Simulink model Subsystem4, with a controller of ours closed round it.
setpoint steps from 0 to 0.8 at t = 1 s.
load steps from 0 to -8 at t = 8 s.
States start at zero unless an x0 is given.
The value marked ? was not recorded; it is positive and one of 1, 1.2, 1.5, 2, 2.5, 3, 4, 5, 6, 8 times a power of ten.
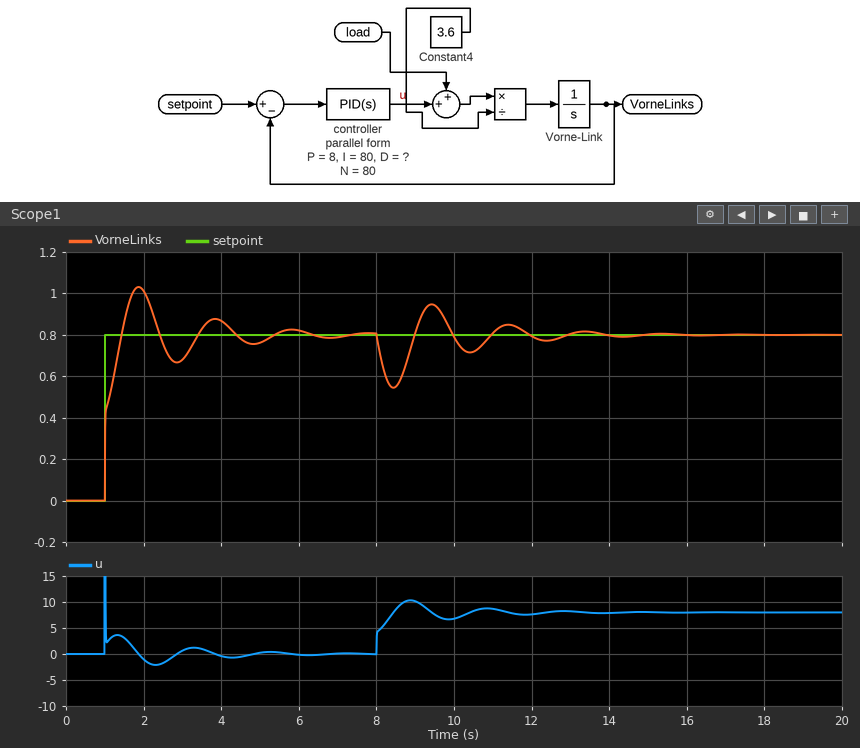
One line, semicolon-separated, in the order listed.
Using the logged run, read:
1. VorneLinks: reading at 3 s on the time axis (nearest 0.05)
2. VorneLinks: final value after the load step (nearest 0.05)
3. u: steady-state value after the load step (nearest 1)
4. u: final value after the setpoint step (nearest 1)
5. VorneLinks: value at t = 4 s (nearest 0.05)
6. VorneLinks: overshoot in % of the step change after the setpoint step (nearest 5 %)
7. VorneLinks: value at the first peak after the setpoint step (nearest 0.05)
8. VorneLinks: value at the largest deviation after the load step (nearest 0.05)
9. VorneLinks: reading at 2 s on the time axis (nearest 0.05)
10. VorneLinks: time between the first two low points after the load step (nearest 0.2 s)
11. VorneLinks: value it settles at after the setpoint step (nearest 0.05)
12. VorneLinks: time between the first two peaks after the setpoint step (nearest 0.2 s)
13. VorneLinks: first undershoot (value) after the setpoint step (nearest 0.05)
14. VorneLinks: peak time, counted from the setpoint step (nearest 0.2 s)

0.70; 0.80; 8; 0; 0.85; 30 %; 1.05; 0.55; 1.00; 2.0 s; 0.80; 2.0 s; 0.65; 0.8 s
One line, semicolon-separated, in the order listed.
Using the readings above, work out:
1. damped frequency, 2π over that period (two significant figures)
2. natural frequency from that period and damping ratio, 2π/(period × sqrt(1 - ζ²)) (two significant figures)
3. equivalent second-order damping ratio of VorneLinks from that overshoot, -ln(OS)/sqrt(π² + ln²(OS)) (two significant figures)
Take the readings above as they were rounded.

3.1 rad/s; 3.4 rad/s; 0.36
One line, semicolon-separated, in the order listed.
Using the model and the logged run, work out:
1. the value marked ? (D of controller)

4
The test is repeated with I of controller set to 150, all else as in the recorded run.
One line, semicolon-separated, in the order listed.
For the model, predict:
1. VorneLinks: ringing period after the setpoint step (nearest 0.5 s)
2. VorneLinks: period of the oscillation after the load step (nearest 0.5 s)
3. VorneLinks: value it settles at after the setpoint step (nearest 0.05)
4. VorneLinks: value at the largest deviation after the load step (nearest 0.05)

1.5 s; 1.5 s; 0.80; 0.60
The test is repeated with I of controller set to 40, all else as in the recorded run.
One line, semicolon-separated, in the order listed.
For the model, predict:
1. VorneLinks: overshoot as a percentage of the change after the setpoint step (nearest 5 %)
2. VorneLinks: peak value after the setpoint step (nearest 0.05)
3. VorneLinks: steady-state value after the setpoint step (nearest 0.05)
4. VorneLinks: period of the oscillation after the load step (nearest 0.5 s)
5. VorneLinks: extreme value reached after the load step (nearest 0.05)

25 %; 1.00; 0.80; 3.0 s; 0.45
